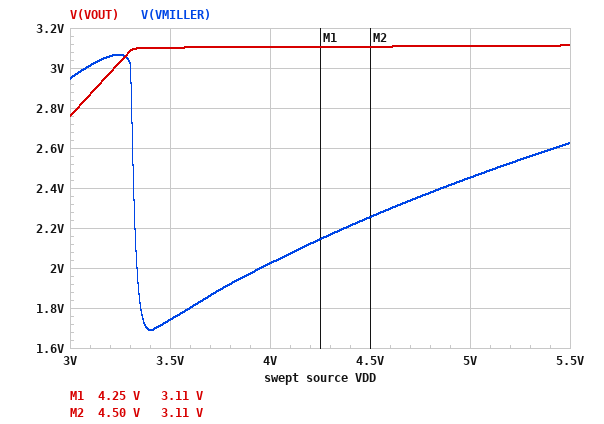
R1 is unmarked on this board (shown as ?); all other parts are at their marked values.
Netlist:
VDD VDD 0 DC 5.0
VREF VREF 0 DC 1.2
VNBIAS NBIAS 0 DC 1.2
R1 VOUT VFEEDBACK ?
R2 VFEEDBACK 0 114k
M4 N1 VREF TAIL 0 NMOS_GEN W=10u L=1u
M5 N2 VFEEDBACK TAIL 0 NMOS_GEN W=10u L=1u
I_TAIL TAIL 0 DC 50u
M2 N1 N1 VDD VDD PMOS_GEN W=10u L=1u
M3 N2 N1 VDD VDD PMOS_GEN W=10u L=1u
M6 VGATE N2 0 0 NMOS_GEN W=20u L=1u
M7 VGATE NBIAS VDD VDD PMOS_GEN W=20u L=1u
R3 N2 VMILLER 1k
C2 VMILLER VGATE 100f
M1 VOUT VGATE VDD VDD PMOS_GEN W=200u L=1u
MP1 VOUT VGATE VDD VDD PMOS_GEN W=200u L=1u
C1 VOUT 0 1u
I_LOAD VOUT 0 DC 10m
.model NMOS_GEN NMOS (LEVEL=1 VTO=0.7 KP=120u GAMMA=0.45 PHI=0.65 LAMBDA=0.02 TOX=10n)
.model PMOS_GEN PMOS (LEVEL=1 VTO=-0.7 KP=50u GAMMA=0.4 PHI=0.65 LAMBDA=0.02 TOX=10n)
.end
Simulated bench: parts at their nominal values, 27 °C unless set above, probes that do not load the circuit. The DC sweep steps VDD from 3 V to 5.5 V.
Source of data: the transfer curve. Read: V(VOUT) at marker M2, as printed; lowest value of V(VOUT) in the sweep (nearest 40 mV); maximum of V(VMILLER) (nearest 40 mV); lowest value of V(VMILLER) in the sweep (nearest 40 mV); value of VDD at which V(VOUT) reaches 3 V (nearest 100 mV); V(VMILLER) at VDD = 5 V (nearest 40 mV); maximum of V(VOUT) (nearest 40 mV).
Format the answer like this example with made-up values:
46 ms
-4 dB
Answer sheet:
3.11 V
2.76 V
3.08 V
1.68 V
3.2 V
2.44 V
3.12 V
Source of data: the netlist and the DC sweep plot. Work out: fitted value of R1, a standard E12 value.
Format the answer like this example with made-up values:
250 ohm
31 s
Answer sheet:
180 kΩ
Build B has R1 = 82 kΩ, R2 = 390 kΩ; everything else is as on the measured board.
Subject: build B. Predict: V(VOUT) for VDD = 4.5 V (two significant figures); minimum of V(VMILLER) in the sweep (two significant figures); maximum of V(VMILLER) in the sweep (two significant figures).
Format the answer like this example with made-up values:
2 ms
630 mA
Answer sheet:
1.5 V
1.4 V
2.6 V
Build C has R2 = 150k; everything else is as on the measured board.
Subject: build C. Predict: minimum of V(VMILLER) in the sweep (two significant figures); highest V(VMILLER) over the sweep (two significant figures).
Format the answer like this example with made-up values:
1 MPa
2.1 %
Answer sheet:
1.4 V
2.6 V
